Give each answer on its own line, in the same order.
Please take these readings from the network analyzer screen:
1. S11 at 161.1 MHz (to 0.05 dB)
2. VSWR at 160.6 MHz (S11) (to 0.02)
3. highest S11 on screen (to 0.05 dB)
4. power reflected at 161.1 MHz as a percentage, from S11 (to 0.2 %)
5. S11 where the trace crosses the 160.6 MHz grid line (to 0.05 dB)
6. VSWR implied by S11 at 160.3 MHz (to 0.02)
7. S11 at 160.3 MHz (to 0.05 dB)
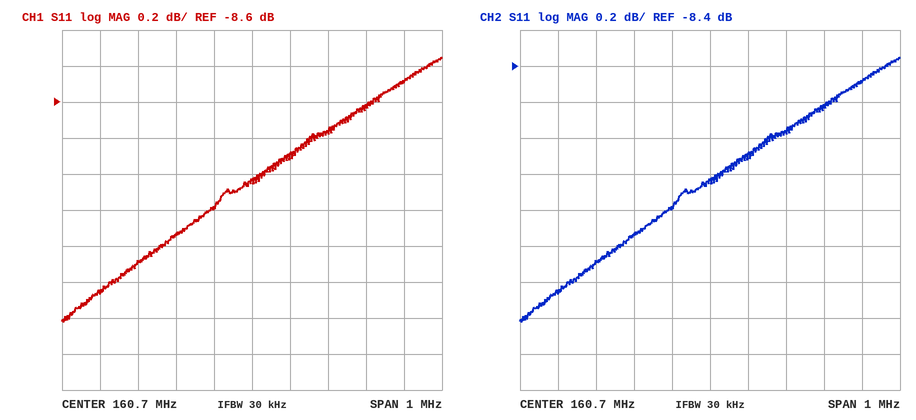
-8.50 dB
2.06
-8.35 dB
14.2 %
-9.20 dB
1.98
-9.65 dB
